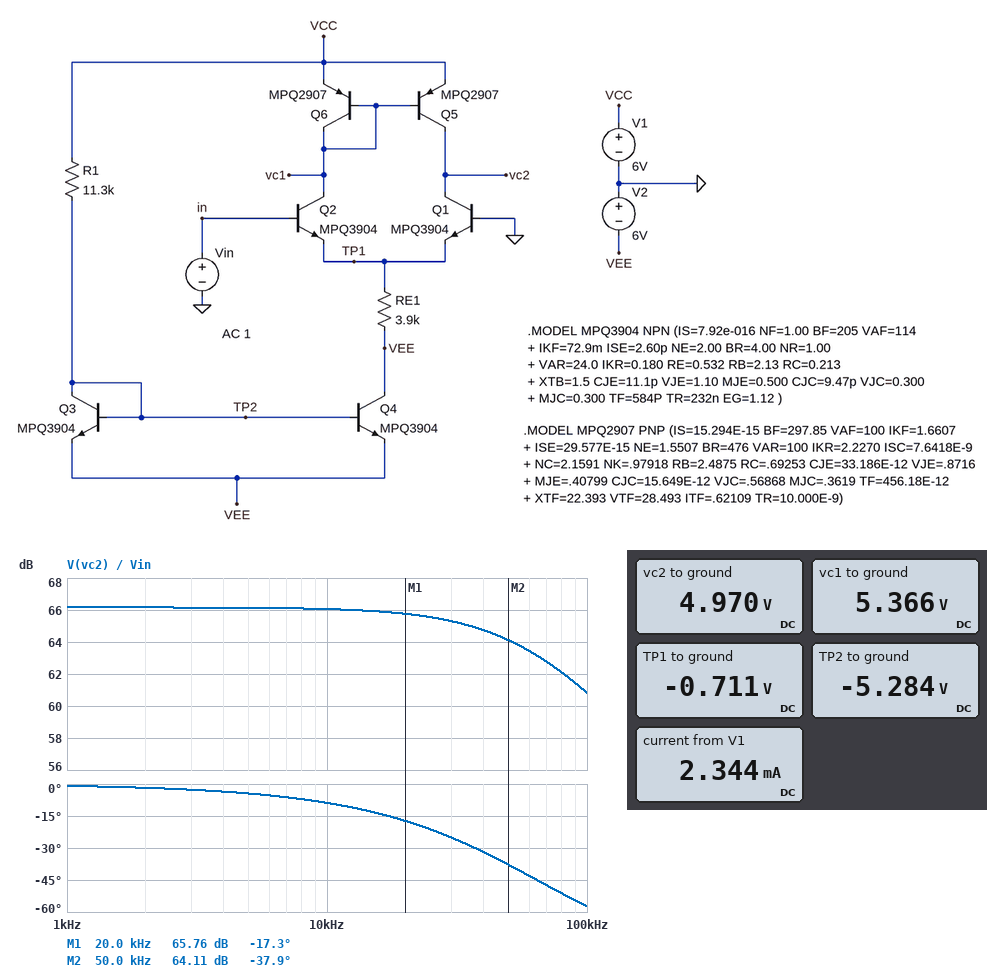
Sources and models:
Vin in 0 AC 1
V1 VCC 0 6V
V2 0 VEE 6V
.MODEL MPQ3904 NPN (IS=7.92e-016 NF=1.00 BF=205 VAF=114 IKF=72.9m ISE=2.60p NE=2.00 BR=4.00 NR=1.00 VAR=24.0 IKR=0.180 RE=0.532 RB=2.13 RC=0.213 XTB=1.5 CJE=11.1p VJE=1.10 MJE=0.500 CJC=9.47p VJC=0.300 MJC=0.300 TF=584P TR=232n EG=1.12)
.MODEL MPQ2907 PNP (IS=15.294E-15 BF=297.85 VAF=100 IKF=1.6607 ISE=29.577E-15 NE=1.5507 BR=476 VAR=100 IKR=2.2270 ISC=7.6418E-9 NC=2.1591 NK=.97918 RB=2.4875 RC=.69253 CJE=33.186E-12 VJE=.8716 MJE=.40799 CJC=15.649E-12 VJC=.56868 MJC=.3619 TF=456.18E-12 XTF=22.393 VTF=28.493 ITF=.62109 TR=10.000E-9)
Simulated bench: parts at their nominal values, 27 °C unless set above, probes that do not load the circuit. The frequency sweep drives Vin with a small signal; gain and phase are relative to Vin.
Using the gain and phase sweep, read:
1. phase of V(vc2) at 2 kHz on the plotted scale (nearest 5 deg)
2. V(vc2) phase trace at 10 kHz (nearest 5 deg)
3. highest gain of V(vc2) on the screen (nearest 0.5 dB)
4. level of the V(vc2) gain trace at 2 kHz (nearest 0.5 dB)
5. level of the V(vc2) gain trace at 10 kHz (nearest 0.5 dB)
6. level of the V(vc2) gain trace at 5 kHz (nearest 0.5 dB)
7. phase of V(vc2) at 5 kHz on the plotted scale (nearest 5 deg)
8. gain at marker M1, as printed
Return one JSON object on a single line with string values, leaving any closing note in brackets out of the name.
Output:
{"phase of V(vc2) at 2 kHz on the plotted scale": "0 deg", "V(vc2) phase trace at 10 kHz": "-10 deg", "highest gain of V(vc2) on the screen": "66.0 dB", "level of the V(vc2) gain trace at 2 kHz": "66.0 dB", "level of the V(vc2) gain trace at 10 kHz": "66.0 dB", "level of the V(vc2) gain trace at 5 kHz": "66.0 dB", "phase of V(vc2) at 5 kHz on the plotted scale": "-5 deg", "gain at marker M1, as printed": "65.76 dB"}
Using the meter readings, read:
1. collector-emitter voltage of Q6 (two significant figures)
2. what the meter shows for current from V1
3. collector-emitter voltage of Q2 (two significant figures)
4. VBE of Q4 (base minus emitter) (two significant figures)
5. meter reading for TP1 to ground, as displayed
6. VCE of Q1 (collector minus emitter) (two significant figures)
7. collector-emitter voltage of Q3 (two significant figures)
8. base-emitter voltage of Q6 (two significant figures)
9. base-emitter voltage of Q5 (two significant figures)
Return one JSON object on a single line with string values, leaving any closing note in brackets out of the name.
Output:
{"collector-emitter voltage of Q6": "-630 mV", "what the meter shows for current from V1": "2.344 mA", "collector-emitter voltage of Q2": "6.1 V", "VBE of Q4 (base minus emitter)": "720 mV", "meter reading for TP1 to ground, as displayed": "-0.711 V", "VCE of Q1 (collector minus emitter)": "5.7 V", "collector-emitter voltage of Q3": "720 mV", "base-emitter voltage of Q6": "-630 mV", "base-emitter voltage of Q5": "-630 mV"}
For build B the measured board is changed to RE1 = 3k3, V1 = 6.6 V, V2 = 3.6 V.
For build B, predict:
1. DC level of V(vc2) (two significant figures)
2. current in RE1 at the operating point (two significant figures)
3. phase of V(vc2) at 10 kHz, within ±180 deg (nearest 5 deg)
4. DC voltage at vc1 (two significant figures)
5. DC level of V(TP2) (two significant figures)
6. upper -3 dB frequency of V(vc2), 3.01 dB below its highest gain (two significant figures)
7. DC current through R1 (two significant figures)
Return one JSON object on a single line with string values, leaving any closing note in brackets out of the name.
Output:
{"DC level of V(vc2)": "5.6 V", "current in RE1 at the operating point": "880 µA", "phase of V(vc2) at 10 kHz, within ±180 deg": "-15 deg", "DC voltage at vc1": "6.0 V", "DC level of V(TP2)": "-2.9 V", "upper -3 dB frequency of V(vc2), 3.01 dB below its highest gain": "42 kHz", "DC current through R1": "840 µA"}
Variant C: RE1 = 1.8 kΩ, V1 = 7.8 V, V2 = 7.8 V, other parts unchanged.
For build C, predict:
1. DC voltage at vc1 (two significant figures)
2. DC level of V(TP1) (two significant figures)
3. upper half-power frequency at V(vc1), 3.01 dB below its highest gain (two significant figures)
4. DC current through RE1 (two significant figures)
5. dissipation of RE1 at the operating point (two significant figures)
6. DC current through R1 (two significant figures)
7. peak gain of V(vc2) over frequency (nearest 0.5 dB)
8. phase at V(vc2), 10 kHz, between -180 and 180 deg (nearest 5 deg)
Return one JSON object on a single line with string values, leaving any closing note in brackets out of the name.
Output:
{"DC voltage at vc1": "7.1 V", "DC level of V(TP1)": "-740 mV", "upper half-power frequency at V(vc1), 3.01 dB below its highest gain": "200 kHz", "DC current through RE1": "3.9 mA", "dissipation of RE1 at the operating point": "28 mW", "DC current through R1": "1.3 mA", "peak gain of V(vc2) over frequency": "66.0 dB", "phase at V(vc2), 10 kHz, between -180 and 180 deg": "-5 deg"}
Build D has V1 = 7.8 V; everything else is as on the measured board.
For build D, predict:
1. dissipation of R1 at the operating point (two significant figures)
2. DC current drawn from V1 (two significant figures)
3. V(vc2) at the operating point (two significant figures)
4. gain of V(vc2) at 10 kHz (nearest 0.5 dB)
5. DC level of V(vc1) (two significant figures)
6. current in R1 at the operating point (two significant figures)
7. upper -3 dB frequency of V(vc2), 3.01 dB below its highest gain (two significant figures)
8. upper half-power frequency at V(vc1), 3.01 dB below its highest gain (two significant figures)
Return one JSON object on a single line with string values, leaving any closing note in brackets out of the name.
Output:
{"dissipation of R1 at the operating point": "15 mW", "DC current drawn from V1": "2.5 mA", "V(vc2) at the operating point": "6.8 V", "gain of V(vc2) at 10 kHz": "66.0 dB", "DC level of V(vc1)": "7.2 V", "current in R1 at the operating point": "1.2 mA", "upper -3 dB frequency of V(vc2), 3.01 dB below its highest gain": "65 kHz", "upper half-power frequency at V(vc1), 3.01 dB below its highest gain": "70 kHz"}
